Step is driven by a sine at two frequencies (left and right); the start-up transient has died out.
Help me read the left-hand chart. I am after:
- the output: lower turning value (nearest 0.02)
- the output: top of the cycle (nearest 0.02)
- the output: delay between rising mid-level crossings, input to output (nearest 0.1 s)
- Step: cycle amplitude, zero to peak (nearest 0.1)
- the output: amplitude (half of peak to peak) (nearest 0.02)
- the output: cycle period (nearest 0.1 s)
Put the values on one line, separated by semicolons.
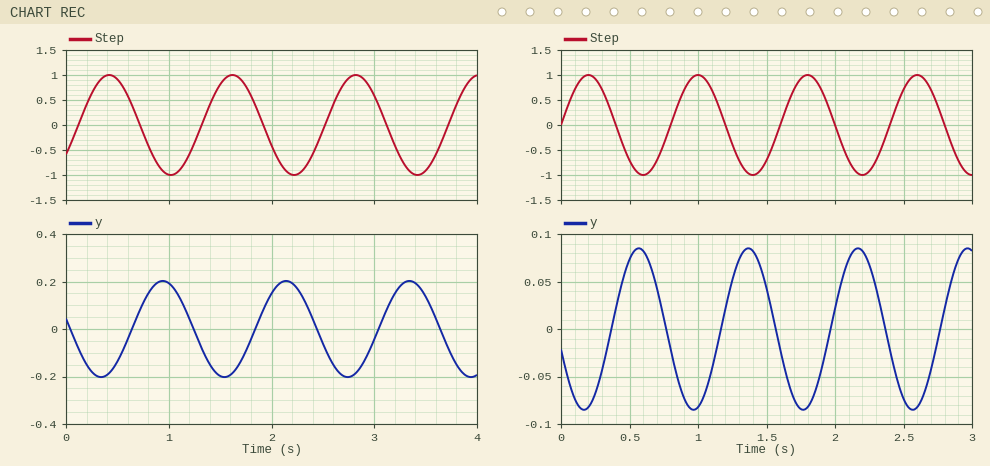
-0.20; 0.20; 0.5 s; 1.0; 0.20; 1.2 s
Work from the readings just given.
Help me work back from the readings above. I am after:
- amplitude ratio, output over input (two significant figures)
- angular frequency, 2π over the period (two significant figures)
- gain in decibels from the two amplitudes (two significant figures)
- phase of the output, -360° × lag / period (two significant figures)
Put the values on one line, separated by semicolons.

0.20; 5.2 rad/s; -14 dB; -150°
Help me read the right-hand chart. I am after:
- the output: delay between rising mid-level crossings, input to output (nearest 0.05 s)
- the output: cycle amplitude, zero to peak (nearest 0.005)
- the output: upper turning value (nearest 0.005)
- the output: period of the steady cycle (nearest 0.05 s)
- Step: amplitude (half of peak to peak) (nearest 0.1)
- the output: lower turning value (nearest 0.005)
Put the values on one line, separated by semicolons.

0.35 s; 0.085; 0.085; 0.80 s; 1.0; -0.085
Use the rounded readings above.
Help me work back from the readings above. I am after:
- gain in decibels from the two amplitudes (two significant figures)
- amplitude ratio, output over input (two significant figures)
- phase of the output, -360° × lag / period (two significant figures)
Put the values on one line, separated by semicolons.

-21 dB; 0.085; -160°
